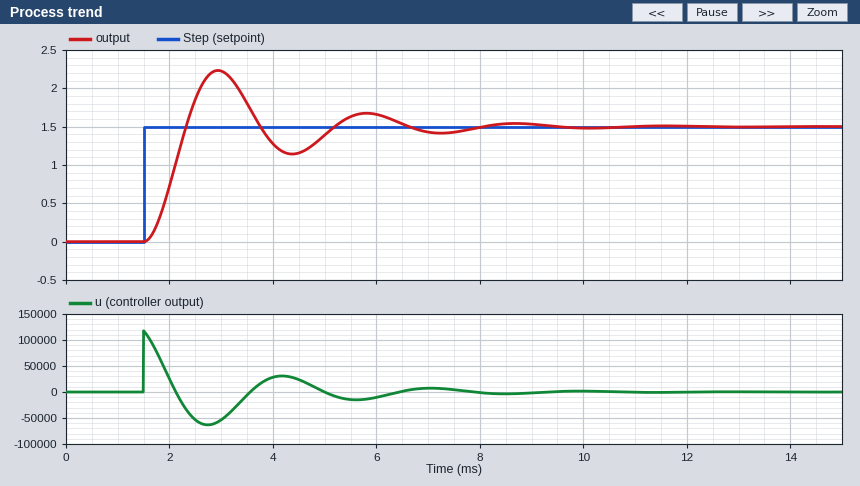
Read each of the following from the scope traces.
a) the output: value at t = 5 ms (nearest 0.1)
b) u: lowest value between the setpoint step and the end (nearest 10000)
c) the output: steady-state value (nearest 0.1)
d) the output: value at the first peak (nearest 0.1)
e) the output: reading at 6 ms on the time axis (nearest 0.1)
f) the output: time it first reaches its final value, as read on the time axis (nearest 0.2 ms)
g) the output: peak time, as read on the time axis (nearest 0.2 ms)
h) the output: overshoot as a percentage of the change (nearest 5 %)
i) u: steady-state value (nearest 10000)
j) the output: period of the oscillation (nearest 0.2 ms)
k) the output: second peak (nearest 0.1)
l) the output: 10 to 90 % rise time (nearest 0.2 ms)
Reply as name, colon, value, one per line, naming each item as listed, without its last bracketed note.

the output: value at t = 5 ms: 1.4
u: lowest value between the setpoint step and the end: -60000
the output: steady-state value: 1.5
the output: value at the first peak: 2.2
the output: reading at 6 ms on the time axis: 1.7
the output: time it first reaches its final value, as read on the time axis: 2.4 ms
the output: peak time, as read on the time axis: 3.0 ms
the output: overshoot as a percentage of the change: 50 %
u: steady-state value: 0
the output: period of the oscillation: 2.8 ms
the output: second peak: 1.7
the output: 10 to 90 % rise time: 0.6 ms
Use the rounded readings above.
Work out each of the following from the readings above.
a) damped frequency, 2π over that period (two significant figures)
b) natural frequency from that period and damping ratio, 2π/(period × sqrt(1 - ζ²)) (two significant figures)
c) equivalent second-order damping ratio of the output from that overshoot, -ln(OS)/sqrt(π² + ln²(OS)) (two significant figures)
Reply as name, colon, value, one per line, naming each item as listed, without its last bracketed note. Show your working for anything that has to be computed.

damped frequency, 2π over that period: 2π / 2.8 = 2.2 rad/ms
natural frequency from that period and damping ratio, 2π/(period × sqrt(1 - ζ²)): 2π / (2.8 × sqrt(1 - 0.22²)) = 2.3 rad/ms
equivalent second-order damping ratio of the output from that overshoot, -ln(OS)/sqrt(π² + ln²(OS)): ln(0.5) = -0.693; 0.693 / sqrt(9.870 + 0.480) = 0.22
